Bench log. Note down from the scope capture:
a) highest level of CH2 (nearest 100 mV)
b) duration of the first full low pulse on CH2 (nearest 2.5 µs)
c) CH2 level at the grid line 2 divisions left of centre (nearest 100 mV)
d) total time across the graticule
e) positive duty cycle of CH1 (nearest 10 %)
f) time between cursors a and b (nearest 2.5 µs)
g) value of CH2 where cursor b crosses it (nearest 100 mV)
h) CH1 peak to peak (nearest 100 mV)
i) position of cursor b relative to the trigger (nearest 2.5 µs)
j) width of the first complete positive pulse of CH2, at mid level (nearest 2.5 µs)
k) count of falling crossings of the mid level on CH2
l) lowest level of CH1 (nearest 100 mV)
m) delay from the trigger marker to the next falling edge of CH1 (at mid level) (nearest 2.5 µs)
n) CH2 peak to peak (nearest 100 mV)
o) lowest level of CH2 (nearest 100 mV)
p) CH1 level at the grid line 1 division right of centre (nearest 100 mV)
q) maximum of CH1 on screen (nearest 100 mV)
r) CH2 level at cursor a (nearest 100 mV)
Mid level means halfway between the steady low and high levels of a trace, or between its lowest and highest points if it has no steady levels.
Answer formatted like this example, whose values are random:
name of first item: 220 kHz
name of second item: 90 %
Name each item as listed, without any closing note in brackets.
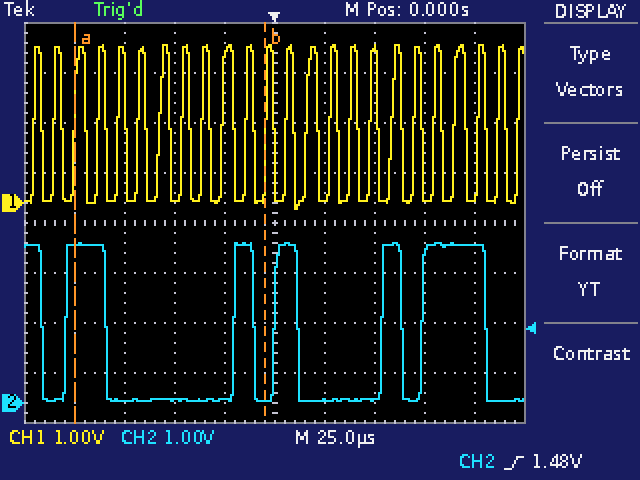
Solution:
highest level of CH2: 3.2 V
duration of the first full low pulse on CH2: 12.5 µs
CH2 level at the grid line 2 divisions left of centre: 100 mV
total time across the graticule: 250 µs
positive duty cycle of CH1: 40 %
time between cursors a and b: 95.0 µs
value of CH2 where cursor b crosses it: 100 mV
CH1 peak to peak: 3.3 V
position of cursor b relative to the trigger: -5.0 µs
width of the first complete positive pulse of CH2, at mid level: 20.0 µs
count of falling crossings of the mid level on CH2: 6
lowest level of CH1: -100 mV
delay from the trigger marker to the next falling edge of CH1 (at mid level): 10.0 µs
CH2 peak to peak: 3.2 V
lowest level of CH2: 0.0 V
CH1 level at the grid line 1 division right of centre: 100 mV
maximum of CH1 on screen: 3.2 V
CH2 level at cursor a: 3.2 V
